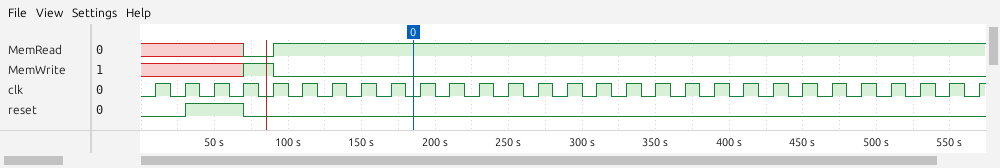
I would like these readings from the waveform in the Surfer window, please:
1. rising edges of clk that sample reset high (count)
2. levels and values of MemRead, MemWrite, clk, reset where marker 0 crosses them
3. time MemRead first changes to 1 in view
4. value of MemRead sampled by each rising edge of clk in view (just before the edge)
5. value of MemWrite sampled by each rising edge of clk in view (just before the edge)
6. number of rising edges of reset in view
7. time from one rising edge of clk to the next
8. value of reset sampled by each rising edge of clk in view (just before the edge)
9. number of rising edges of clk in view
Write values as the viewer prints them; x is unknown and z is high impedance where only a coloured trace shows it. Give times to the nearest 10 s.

2
MemRead=1, MemWrite=0, clk=0, reset=0
90 s
x x x x 0 1 1 1 1 1 1 1 1 1 1 1 1 1 1 1 1 1 1 1 1 1 1 1 1
x x x x 1 0 0 0 0 0 0 0 0 0 0 0 0 0 0 0 0 0 0 0 0 0 0 0 0
1
20 s
0 0 1 1 0 0 0 0 0 0 0 0 0 0 0 0 0 0 0 0 0 0 0 0 0 0 0 0 0
29
